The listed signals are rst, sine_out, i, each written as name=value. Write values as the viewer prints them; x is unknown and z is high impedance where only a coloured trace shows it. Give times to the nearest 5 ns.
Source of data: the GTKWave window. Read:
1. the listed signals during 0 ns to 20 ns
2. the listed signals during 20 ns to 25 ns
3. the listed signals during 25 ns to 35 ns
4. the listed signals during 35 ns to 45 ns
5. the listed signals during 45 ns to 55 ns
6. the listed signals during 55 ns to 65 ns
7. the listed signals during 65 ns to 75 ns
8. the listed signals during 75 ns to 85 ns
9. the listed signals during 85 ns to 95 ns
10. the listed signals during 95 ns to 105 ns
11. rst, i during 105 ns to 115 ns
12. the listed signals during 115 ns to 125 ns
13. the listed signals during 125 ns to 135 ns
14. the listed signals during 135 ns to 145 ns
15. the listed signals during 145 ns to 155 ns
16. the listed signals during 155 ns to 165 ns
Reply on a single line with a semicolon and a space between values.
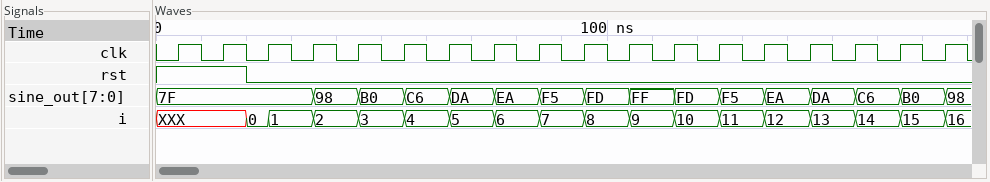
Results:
rst=1, sine_out=7F, i=XXX; rst=0, sine_out=7F, i=0; rst=0, sine_out=7F, i=1; rst=0, sine_out=98, i=2; rst=0, sine_out=B0, i=3; rst=0, sine_out=C6, i=4; rst=0, sine_out=DA, i=5; rst=0, sine_out=EA, i=6; rst=0, sine_out=F5, i=7; rst=0, sine_out=FD, i=8; rst=0, i=9; rst=0, sine_out=FD, i=10; rst=0, sine_out=F5, i=11; rst=0, sine_out=EA, i=12; rst=0, sine_out=DA, i=13; rst=0, sine_out=C6, i=14
